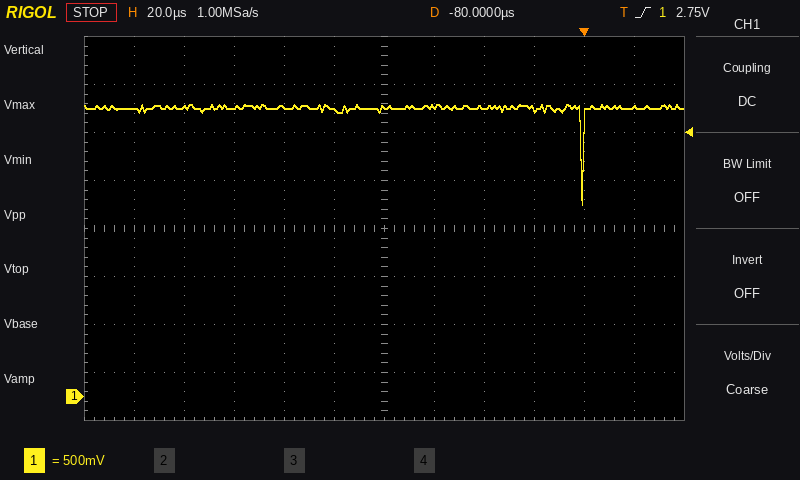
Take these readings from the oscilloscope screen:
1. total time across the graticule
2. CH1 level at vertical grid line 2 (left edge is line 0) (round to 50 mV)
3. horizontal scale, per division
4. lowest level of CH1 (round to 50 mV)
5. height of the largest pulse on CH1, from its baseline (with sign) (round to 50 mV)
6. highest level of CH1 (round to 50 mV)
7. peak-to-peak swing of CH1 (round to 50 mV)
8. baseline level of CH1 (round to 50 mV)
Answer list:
240 µs
3.00 V
20 µs
2.00 V
-1.00 V
3.05 V
1.05 V
3.00 V
